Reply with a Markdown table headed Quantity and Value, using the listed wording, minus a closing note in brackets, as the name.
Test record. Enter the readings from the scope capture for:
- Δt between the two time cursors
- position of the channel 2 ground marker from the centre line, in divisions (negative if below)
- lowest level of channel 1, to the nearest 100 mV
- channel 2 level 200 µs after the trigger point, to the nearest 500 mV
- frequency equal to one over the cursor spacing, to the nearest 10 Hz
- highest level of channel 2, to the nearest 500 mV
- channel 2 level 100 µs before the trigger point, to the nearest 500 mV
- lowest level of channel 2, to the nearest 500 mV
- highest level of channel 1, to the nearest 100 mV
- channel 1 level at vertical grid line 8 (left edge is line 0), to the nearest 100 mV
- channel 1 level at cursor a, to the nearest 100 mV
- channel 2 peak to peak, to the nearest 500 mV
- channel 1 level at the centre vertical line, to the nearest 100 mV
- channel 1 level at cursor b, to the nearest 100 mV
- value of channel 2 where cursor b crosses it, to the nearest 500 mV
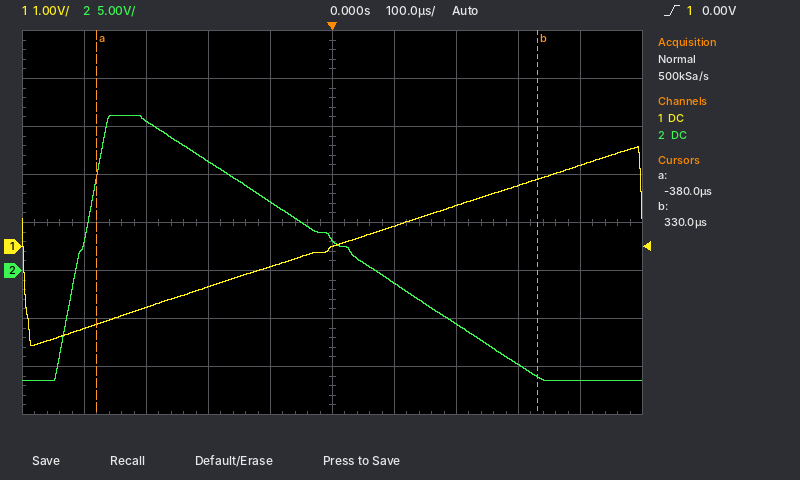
| Quantity | Value |
|---|---|
| Δt between the two time cursors | 710 µs |
| position of the channel 2 ground marker from the centre line, in divisions | -1.0 div |
| lowest level of channel 1, to the nearest 100 mV | -2.1 V |
| channel 2 level 200 µs after the trigger point, to the nearest 500 mV | -5.5 V |
| frequency equal to one over the cursor spacing, to the nearest 10 Hz | 1.41 kHz |
| highest level of channel 2, to the nearest 500 mV | 16.0 V |
| channel 2 level 100 µs before the trigger point, to the nearest 500 mV | 7.0 V |
| lowest level of channel 2, to the nearest 500 mV | -11.5 V |
| highest level of channel 1, to the nearest 100 mV | 2.1 V |
| channel 1 level at vertical grid line 8 (left edge is line 0), to the nearest 100 mV | 1.3 V |
| channel 1 level at cursor a, to the nearest 100 mV | -1.6 V |
| channel 2 peak to peak, to the nearest 500 mV | 27.5 V |
| channel 1 level at the centre vertical line, to the nearest 100 mV | 0.0 V |
| channel 1 level at cursor b, to the nearest 100 mV | 1.4 V |
| value of channel 2 where cursor b crosses it, to the nearest 500 mV | -11.0 V |
